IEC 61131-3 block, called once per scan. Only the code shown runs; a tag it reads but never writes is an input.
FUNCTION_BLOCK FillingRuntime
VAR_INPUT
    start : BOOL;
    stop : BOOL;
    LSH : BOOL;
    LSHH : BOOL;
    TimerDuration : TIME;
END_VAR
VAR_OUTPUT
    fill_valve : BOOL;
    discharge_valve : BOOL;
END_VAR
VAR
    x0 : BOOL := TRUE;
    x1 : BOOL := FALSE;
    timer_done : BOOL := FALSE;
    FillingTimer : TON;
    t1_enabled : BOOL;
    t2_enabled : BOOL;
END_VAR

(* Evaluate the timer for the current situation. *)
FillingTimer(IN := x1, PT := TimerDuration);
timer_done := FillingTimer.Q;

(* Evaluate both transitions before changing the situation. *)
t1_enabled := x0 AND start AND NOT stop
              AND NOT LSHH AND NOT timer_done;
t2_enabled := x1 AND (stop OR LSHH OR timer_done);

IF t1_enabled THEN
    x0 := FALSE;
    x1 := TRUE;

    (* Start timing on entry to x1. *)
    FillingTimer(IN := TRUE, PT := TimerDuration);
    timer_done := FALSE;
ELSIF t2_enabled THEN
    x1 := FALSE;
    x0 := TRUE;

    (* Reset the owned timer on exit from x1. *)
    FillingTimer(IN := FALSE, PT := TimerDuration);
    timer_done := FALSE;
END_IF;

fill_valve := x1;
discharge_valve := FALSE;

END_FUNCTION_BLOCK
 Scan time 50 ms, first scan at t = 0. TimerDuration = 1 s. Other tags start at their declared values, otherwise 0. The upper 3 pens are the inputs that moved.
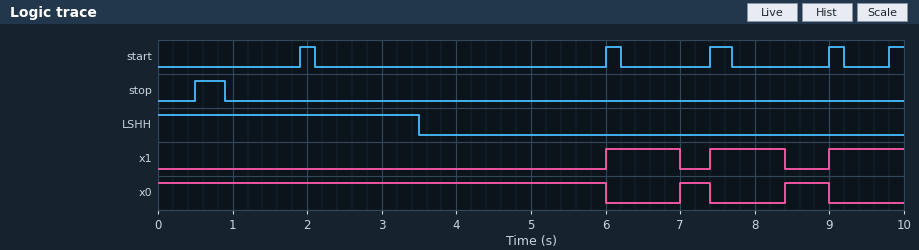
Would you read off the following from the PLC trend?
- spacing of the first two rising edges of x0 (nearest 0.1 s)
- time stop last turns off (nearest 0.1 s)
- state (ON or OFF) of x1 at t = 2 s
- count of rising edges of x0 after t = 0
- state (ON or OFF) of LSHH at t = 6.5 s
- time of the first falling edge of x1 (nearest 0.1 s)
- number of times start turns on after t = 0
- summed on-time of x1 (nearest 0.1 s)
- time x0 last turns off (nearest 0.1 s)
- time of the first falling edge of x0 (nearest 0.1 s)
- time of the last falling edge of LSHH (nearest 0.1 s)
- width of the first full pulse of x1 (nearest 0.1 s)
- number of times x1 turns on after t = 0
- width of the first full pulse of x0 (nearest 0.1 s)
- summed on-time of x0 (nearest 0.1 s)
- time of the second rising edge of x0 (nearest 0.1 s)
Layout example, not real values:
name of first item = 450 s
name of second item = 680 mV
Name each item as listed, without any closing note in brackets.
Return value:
spacing of the first two rising edges of x0 = 1.4 s
time stop last turns off = 0.9 s
state (ON or OFF) of x1 at t = 2 s = OFF
count of rising edges of x0 after t = 0 = 2
state (ON or OFF) of LSHH at t = 6.5 s = OFF
time of the first falling edge of x1 = 7.0 s
number of times start turns on after t = 0 = 5
summed on-time of x1 = 3.0 s
time x0 last turns off = 9.0 s
time of the first falling edge of x0 = 6.0 s
time of the last falling edge of LSHH = 3.5 s
width of the first full pulse of x1 = 1.0 s
number of times x1 turns on after t = 0 = 3
width of the first full pulse of x0 = 0.4 s
summed on-time of x0 = 7.0 s
time of the second rising edge of x0 = 8.4 s
